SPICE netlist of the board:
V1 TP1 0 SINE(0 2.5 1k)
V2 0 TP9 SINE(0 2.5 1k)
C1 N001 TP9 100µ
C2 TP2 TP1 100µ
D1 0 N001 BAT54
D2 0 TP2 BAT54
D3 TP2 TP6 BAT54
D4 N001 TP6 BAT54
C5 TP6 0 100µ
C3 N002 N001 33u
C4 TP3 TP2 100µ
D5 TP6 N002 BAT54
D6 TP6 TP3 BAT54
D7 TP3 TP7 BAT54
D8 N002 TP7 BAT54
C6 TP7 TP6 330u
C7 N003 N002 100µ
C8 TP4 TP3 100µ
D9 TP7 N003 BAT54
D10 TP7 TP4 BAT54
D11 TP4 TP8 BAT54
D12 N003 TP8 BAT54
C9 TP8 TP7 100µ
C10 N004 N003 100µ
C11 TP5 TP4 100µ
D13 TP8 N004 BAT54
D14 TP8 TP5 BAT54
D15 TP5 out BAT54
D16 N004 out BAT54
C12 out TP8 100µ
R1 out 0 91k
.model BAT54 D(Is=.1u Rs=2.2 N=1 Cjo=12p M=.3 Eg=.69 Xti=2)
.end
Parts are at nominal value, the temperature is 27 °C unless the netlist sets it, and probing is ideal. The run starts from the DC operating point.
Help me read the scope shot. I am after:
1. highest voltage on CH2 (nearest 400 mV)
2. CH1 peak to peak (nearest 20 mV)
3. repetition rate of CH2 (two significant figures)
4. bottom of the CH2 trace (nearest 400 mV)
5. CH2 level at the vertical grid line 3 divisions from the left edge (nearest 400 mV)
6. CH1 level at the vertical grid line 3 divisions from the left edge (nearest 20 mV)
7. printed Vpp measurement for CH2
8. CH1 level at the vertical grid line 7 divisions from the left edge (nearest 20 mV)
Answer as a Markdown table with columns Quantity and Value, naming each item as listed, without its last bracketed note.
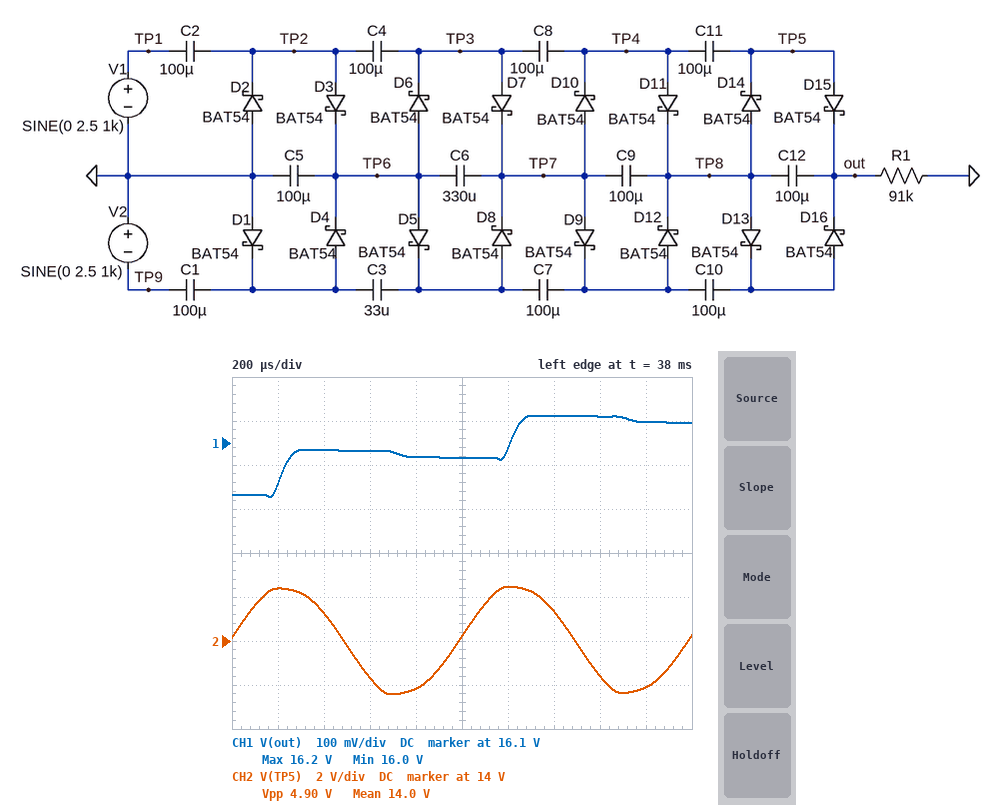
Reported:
| Quantity | Value |
|---|---|
| highest voltage on CH2 | 16.4 V |
| CH1 peak to peak | 180 mV |
| repetition rate of CH2 | 1.0 kHz |
| bottom of the CH2 trace | 11.6 V |
| CH2 level at the vertical grid line 3 divisions from the left edge | 12.4 V |
| CH1 level at the vertical grid line 3 divisions from the left edge | 16.08 V |
| printed Vpp measurement for CH2 | 4.90 V |
| CH1 level at the vertical grid line 7 divisions from the left edge | 16.16 V |
